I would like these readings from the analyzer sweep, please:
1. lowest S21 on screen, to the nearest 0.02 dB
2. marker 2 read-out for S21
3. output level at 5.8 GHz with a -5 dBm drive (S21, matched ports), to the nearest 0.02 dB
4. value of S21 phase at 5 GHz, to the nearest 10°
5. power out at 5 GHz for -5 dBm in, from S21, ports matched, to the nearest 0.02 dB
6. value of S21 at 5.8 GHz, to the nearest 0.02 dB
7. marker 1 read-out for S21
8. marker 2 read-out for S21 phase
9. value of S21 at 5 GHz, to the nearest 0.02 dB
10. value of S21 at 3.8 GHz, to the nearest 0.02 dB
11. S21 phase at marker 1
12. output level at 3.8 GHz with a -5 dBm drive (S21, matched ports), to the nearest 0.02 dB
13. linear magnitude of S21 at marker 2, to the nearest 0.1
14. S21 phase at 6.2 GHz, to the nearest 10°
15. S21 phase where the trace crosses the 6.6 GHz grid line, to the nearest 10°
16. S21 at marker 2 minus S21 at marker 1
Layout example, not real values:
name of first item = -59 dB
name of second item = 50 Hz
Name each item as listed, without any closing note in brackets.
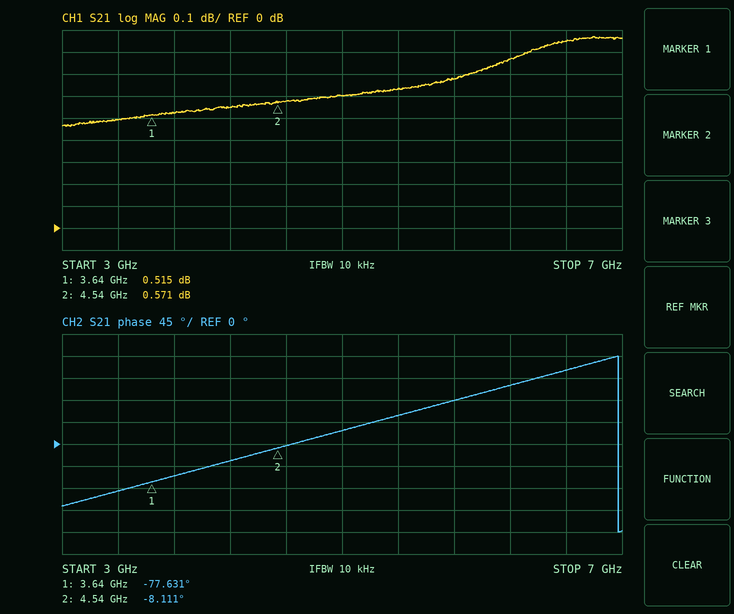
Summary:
lowest S21 on screen, to the nearest 0.02 dB = 0.46 dB
marker 2 read-out for S21 = 0.571 dB
output level at 5.8 GHz with a -5 dBm drive (S21, matched ports), to the nearest 0.02 dB = -4.32 dBm
value of S21 phase at 5 GHz, to the nearest 10° = 30°
power out at 5 GHz for -5 dBm in, from S21, ports matched, to the nearest 0.02 dB = -4.40 dBm
value of S21 at 5.8 GHz, to the nearest 0.02 dB = 0.68 dB
marker 1 read-out for S21 = 0.515 dB
marker 2 read-out for S21 phase = -8.111°
value of S21 at 5 GHz, to the nearest 0.02 dB = 0.60 dB
value of S21 at 3.8 GHz, to the nearest 0.02 dB = 0.52 dB
S21 phase at marker 1 = -77.631°
output level at 3.8 GHz with a -5 dBm drive (S21, matched ports), to the nearest 0.02 dB = -4.48 dBm
linear magnitude of S21 at marker 2, to the nearest 0.1 = 1.1
S21 phase at 6.2 GHz, to the nearest 10° = 120°
S21 phase where the trace crosses the 6.6 GHz grid line, to the nearest 10° = 150°
S21 at marker 2 minus S21 at marker 1 = 0.056 dB
